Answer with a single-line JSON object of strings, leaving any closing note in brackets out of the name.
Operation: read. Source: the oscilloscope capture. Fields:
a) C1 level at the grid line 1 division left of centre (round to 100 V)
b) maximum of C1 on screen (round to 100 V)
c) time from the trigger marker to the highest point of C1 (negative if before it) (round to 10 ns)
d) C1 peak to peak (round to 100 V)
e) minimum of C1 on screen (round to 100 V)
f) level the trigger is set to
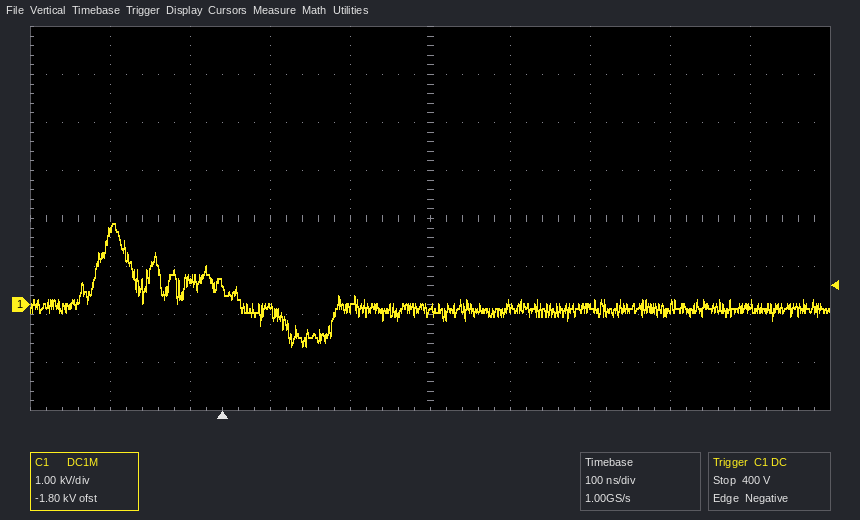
{"C1 level at the grid line 1 division left of centre": "-100 V", "maximum of C1 on screen": "1.7 kV", "time from the trigger marker to the highest point of C1 (negative if before it)": "-140 ns", "C1 peak to peak": "2.6 kV", "minimum of C1 on screen": "-900 V", "level the trigger is set to": "400 V"}
